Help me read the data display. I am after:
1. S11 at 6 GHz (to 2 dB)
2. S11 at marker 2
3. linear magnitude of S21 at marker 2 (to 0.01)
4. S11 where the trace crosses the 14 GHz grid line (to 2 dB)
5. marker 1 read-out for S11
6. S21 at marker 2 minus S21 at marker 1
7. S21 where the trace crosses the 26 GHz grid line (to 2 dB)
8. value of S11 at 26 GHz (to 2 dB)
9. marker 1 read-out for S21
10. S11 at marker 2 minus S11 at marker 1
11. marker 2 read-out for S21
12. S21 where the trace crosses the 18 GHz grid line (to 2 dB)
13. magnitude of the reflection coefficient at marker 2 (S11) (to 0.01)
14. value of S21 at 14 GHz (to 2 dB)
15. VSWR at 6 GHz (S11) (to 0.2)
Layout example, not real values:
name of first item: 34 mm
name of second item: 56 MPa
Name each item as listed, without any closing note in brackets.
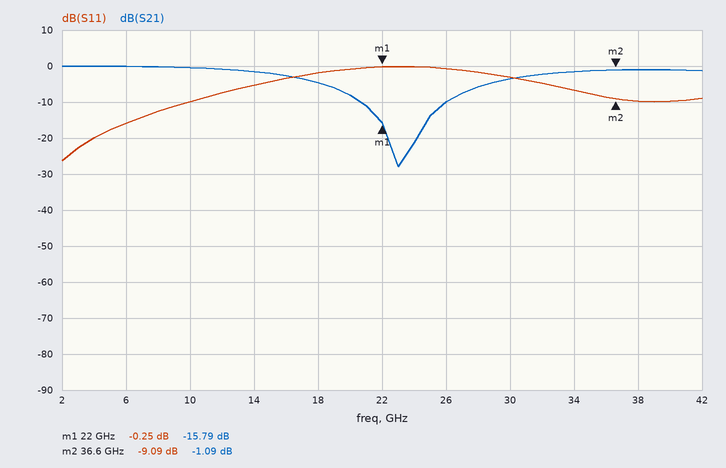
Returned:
S11 at 6 GHz: -16 dB
S11 at marker 2: -9.09 dB
linear magnitude of S21 at marker 2: 0.88
S11 where the trace crosses the 14 GHz grid line: -6 dB
marker 1 read-out for S11: -0.25 dB
S21 at marker 2 minus S21 at marker 1: 14.70 dB
S21 where the trace crosses the 26 GHz grid line: -10 dB
value of S11 at 26 GHz: 0 dB
marker 1 read-out for S21: -15.79 dB
S11 at marker 2 minus S11 at marker 1: -8.84 dB
marker 2 read-out for S21: -1.09 dB
S21 where the trace crosses the 18 GHz grid line: -4 dB
magnitude of the reflection coefficient at marker 2 (S11): 0.35
value of S21 at 14 GHz: -2 dB
VSWR at 6 GHz (S11): 1.4
